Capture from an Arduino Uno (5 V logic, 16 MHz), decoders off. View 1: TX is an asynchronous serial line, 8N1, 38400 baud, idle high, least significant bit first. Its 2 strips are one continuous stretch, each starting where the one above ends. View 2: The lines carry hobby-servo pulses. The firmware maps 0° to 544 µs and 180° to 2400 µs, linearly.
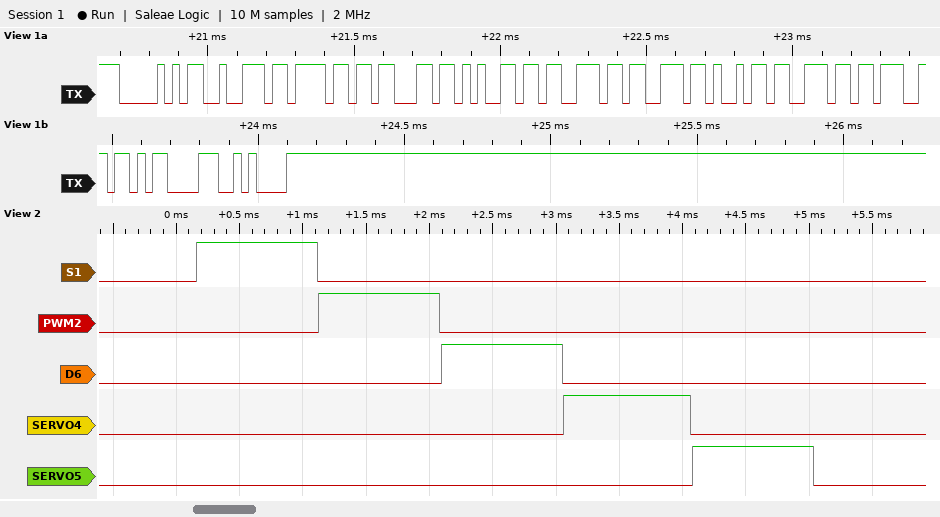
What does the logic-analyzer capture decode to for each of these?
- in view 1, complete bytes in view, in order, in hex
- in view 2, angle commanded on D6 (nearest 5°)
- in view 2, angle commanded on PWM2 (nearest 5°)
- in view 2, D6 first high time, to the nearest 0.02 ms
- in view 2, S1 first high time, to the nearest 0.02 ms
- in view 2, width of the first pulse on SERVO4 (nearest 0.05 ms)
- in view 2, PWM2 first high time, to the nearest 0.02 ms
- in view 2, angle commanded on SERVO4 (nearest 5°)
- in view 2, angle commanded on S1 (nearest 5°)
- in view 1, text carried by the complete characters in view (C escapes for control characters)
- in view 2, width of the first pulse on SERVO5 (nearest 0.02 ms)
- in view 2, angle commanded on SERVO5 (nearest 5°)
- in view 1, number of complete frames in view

50 72 6F 63 65 73 73 69 6E 67 0D 0A
40°
40°
0.96 ms
0.96 ms
1.00 ms
0.96 ms
45°
40°
"Processing\r\n"
0.96 ms
40°
12
